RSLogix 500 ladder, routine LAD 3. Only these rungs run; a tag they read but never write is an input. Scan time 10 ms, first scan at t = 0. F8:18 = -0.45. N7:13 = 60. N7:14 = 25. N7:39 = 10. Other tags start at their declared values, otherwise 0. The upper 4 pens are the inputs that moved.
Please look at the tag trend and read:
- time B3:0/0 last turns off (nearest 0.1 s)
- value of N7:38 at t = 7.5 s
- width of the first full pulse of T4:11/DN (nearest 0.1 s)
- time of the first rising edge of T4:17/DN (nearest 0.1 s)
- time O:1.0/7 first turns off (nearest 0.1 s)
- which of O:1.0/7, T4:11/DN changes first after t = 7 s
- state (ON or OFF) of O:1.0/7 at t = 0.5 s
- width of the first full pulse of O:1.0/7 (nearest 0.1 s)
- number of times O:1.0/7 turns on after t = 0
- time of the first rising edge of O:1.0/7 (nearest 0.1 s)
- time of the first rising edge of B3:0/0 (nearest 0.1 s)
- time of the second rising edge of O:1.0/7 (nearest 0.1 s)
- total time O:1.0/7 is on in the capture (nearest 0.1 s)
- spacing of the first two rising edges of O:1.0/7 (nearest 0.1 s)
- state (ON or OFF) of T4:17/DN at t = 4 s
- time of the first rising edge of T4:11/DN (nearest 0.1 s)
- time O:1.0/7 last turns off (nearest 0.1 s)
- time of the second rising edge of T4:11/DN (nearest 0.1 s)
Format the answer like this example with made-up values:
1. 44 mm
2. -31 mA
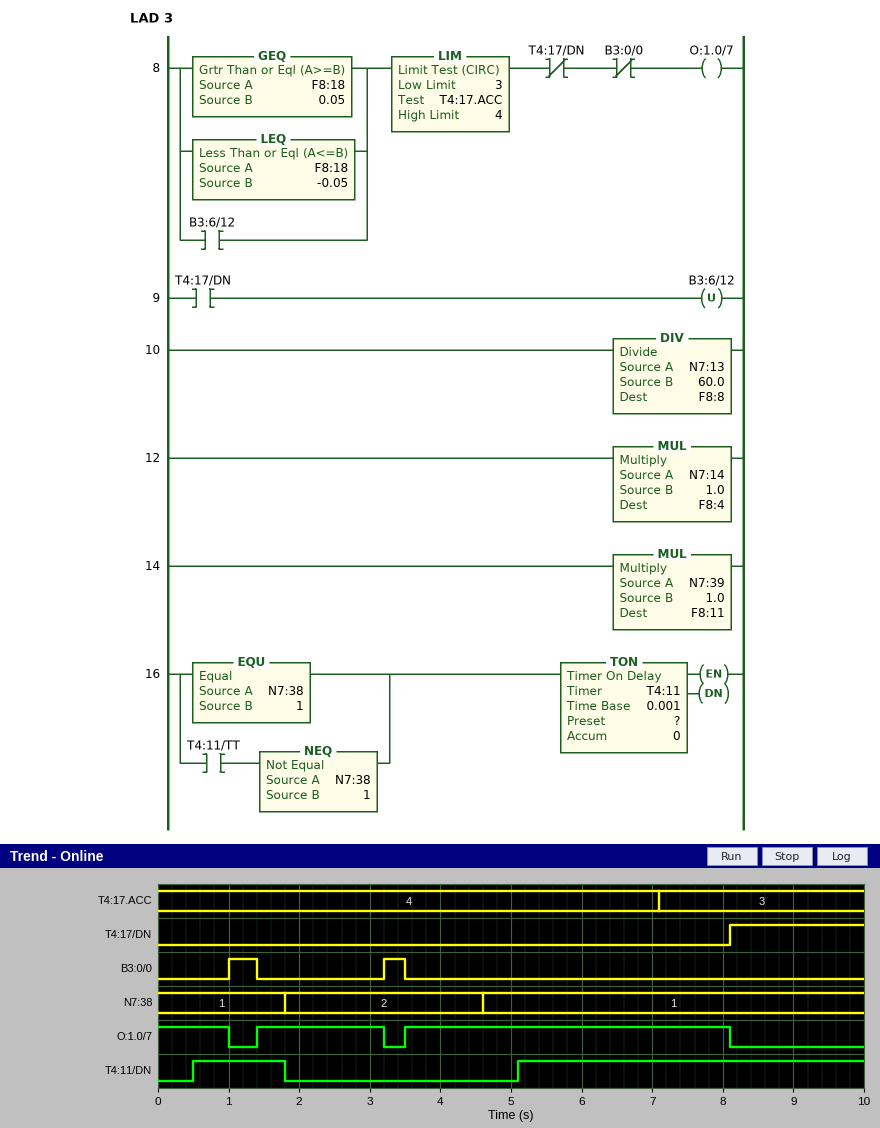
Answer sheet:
1. 3.5 s
2. 1
3. 1.3 s
4. 8.1 s
5. 1.0 s
6. O:1.0/7
7. ON
8. 1.8 s
9. 2
10. 1.4 s
11. 1.0 s
12. 3.5 s
13. 7.4 s
14. 2.1 s
15. OFF
16. 0.5 s
17. 8.1 s
18. 5.1 s
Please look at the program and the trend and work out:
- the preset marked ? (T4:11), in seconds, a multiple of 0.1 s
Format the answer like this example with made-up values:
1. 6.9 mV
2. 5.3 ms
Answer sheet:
1. 0.5 s
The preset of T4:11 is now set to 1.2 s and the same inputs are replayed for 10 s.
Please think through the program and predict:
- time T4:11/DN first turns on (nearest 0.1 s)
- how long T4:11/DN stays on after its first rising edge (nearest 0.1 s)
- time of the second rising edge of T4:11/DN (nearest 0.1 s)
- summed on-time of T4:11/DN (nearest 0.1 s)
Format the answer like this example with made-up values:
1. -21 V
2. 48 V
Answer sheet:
1. 1.2 s
2. 0.6 s
3. 5.8 s
4. 4.8 s
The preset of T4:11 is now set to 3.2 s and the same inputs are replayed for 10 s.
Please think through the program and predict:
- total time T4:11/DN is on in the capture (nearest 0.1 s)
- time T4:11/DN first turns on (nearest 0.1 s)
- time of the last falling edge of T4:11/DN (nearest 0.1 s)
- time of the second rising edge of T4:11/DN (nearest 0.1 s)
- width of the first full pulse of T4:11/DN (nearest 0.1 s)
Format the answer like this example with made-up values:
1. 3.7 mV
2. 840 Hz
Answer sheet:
1. 2.2 s
2. 3.2 s
3. 3.2 s
4. 7.8 s
5. 0.0 s
